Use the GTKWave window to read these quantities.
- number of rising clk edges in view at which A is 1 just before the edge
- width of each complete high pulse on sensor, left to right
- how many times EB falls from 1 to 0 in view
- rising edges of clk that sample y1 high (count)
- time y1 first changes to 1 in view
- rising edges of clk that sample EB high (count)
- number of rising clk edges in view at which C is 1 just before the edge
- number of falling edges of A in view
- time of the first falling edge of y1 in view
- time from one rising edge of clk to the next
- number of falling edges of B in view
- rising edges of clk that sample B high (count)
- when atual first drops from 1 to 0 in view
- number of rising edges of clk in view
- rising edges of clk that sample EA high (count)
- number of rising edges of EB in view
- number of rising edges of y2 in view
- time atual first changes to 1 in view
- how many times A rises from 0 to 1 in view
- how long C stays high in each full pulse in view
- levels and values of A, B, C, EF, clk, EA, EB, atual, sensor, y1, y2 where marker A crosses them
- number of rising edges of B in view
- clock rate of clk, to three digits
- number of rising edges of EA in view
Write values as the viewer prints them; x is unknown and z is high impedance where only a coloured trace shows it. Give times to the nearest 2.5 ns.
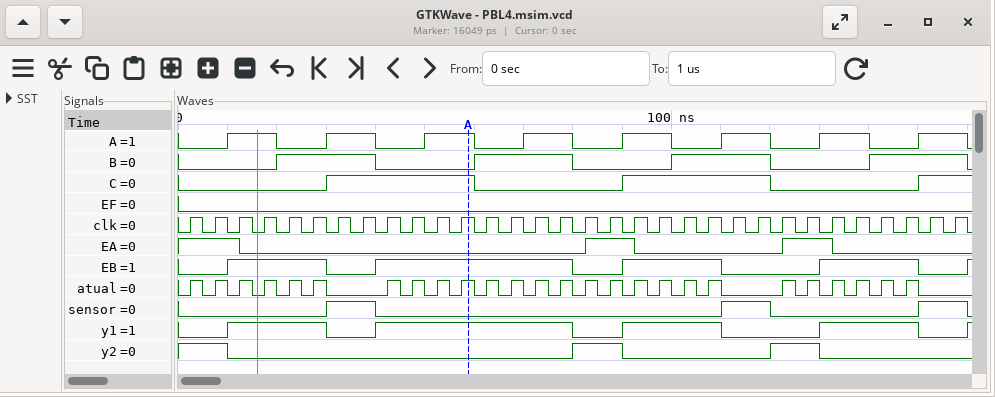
16
10 ns, 10 ns, 10 ns
4
20
10 ns
20
14
8
30 ns
5 ns
4
16
5 ns
32
7
5
2
2.5 ns
8
30 ns, 30 ns
A=1, B=0, C=1, EF=0, clk=1, EA=0, EB=1, atual=1, sensor=0, y1=1, y2=0
4
200 MHz
2
